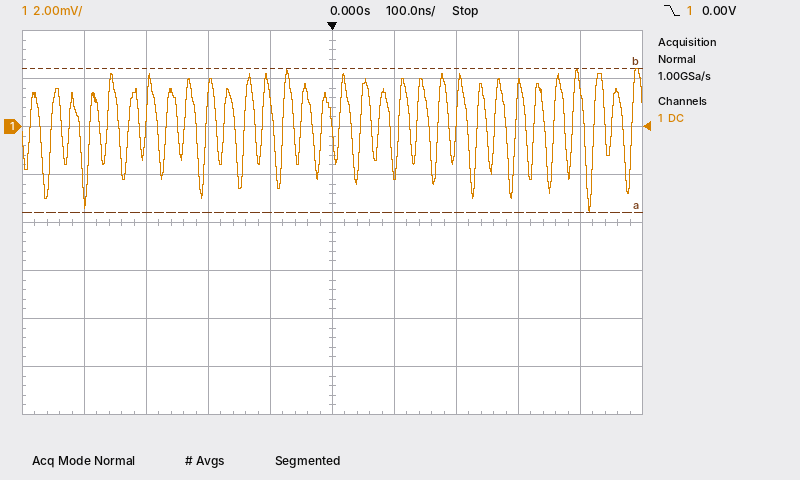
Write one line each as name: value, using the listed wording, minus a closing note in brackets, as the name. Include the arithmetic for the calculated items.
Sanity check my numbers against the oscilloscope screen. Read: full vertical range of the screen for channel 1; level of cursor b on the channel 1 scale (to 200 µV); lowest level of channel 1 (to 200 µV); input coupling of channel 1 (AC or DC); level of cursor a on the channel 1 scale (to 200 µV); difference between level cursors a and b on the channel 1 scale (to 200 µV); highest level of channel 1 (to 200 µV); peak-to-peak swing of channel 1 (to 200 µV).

full vertical range of the screen for channel 1: 16 mV
level of cursor b on the channel 1 scale: 2.4 mV
lowest level of channel 1: -3.6 mV
input coupling of channel 1: DC
level of cursor a on the channel 1 scale: -3.6 mV
difference between level cursors a and b on the channel 1 scale: 6.0 mV
highest level of channel 1: 2.4 mV
peak-to-peak swing of channel 1: 2.4 mV − (-3.6 mV) = 6.0 mV
